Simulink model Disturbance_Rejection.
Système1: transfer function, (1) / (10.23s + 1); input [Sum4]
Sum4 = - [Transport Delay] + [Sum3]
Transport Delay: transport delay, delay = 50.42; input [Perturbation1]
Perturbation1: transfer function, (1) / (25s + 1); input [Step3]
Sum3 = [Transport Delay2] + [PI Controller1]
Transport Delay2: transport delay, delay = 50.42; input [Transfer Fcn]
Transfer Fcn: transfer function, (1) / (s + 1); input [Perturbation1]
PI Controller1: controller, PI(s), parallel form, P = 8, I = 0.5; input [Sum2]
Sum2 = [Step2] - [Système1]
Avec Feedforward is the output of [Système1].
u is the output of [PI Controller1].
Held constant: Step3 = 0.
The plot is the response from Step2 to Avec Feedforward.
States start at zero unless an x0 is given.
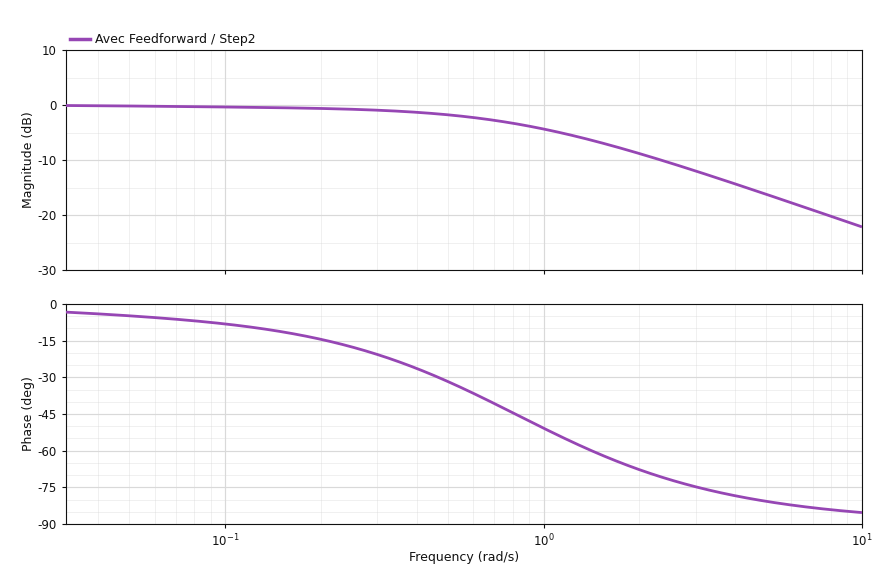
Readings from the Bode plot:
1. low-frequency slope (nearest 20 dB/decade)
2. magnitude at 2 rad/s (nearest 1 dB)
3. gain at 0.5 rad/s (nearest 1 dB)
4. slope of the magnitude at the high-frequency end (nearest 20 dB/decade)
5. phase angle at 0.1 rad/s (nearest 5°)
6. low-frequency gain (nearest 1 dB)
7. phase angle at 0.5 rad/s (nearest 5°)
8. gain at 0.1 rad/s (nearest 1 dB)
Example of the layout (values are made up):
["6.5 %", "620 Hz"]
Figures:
["0 dB/decade", "-9 dB", "-2 dB", "-20 dB/decade", "-10°", "0 dB", "-30°", "0 dB"]
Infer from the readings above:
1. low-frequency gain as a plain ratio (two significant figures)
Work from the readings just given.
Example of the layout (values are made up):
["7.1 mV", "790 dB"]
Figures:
["1.0"]
